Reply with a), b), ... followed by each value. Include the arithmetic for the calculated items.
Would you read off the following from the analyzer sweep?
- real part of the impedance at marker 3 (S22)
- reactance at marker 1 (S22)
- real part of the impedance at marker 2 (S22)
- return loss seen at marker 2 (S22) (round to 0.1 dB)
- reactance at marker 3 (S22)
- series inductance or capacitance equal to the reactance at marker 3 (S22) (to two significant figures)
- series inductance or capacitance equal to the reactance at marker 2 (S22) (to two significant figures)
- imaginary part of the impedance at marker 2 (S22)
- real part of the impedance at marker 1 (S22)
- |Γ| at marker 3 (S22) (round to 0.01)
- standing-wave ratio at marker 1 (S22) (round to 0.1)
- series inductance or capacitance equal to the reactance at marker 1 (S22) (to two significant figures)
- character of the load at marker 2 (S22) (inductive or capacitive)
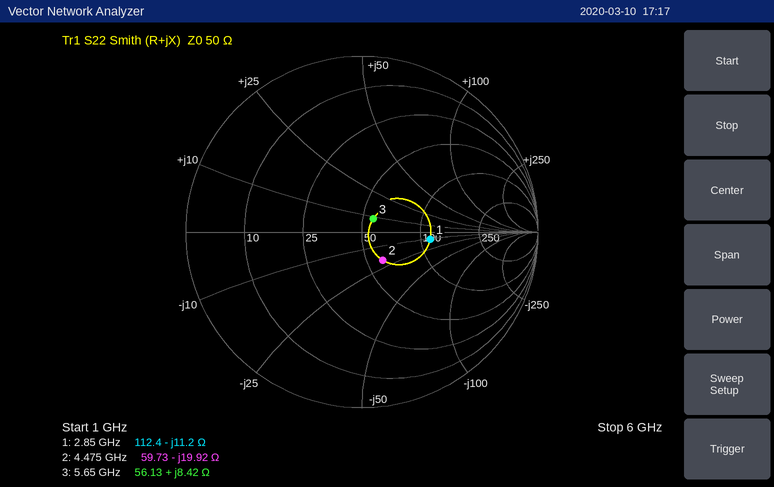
a) 56.13 Ω
b) -11.2 Ω
c) 59.73 Ω
d) 14.0 dB
e) +8.42 Ω
f) L = 8.42 Ω/(2π × 5.65 GHz) ≈ 237 pH, so 240 pH to two significant figures
g) C = 1/(2π × 4.475 GHz × 19.92 Ω) ≈ 1.8 pF
h) -19.92 Ω
i) 112.4 Ω
j) 0.10
k) 2.3
l) C = 1/(2π × 2.85 GHz × 11.2 Ω) ≈ 5.0 pF
m) capacitive
